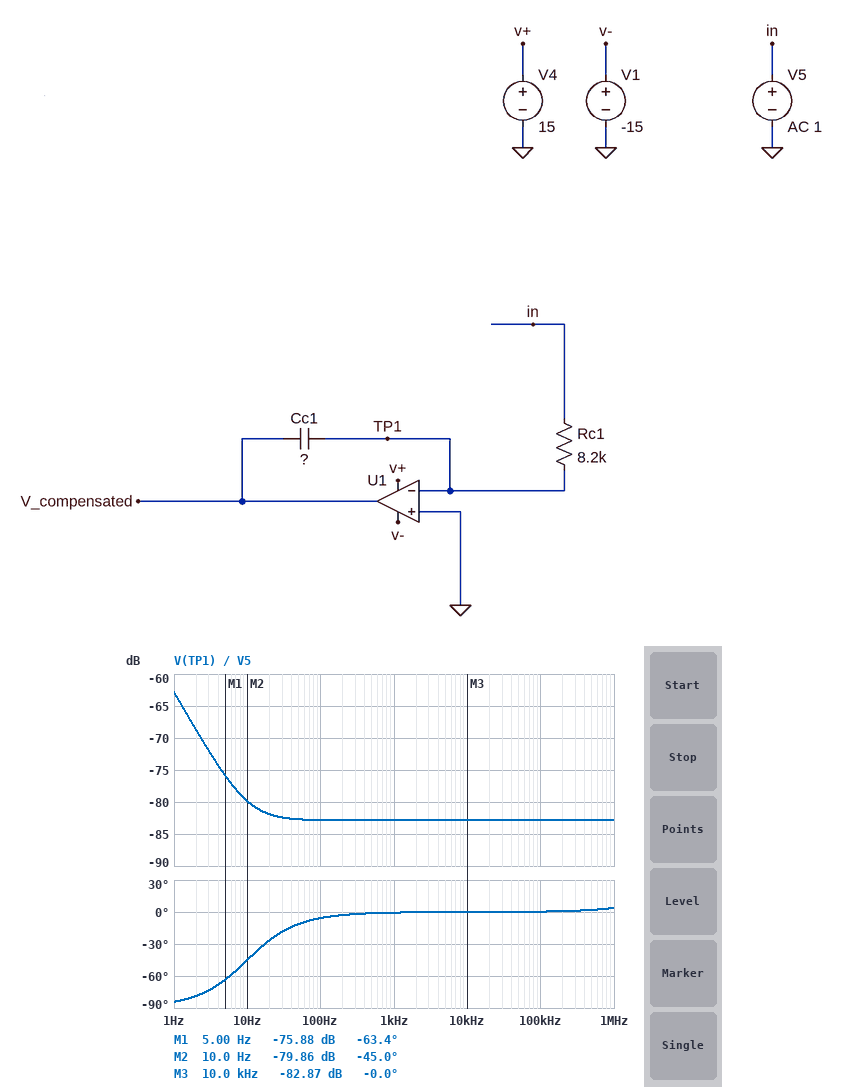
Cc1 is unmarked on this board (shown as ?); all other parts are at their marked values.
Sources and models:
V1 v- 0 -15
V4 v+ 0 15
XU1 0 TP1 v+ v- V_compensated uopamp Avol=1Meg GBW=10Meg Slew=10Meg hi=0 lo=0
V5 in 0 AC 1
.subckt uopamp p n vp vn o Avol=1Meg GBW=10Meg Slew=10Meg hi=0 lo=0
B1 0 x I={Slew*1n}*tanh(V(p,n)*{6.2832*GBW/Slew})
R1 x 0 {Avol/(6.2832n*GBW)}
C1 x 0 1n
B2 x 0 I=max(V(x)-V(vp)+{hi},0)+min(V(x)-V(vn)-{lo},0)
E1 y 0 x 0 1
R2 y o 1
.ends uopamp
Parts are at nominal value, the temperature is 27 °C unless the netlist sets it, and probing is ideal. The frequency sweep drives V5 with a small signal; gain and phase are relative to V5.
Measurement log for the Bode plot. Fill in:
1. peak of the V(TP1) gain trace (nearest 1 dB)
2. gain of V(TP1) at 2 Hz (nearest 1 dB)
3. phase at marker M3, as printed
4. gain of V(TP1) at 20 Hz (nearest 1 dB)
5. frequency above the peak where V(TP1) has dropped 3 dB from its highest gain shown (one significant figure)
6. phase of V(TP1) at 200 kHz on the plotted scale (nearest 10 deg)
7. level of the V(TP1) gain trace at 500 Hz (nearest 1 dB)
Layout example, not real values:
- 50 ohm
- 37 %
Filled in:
- -63 dB
- -69 dB
- -0.0 deg
- -82 dB
- 1 Hz
- 0 deg
- -83 dB
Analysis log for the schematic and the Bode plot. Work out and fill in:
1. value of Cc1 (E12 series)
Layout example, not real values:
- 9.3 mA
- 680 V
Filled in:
- 27 nF
